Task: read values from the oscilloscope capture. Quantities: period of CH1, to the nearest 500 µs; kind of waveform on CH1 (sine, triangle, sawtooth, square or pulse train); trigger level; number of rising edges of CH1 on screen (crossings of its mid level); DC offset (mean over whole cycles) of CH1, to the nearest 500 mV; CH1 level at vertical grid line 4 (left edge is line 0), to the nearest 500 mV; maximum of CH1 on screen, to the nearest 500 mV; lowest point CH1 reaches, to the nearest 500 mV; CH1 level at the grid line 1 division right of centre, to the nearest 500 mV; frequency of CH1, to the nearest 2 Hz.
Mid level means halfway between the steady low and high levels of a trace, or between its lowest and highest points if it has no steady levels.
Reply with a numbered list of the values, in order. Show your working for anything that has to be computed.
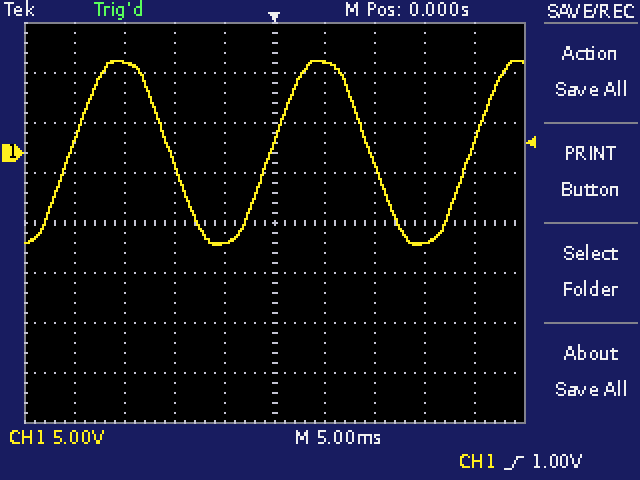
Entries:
1. 20.0 ms
2. sine
3. 1.00 V
4. 3
5. (9.0 V + (-9.0 V)) / 2 ≈ 0.0 V
6. -9.0 V
7. 9.0 V
8. -9.0 V
9. 9.0 V
10. 1 / 20.0 ms ≈ 50 Hz
